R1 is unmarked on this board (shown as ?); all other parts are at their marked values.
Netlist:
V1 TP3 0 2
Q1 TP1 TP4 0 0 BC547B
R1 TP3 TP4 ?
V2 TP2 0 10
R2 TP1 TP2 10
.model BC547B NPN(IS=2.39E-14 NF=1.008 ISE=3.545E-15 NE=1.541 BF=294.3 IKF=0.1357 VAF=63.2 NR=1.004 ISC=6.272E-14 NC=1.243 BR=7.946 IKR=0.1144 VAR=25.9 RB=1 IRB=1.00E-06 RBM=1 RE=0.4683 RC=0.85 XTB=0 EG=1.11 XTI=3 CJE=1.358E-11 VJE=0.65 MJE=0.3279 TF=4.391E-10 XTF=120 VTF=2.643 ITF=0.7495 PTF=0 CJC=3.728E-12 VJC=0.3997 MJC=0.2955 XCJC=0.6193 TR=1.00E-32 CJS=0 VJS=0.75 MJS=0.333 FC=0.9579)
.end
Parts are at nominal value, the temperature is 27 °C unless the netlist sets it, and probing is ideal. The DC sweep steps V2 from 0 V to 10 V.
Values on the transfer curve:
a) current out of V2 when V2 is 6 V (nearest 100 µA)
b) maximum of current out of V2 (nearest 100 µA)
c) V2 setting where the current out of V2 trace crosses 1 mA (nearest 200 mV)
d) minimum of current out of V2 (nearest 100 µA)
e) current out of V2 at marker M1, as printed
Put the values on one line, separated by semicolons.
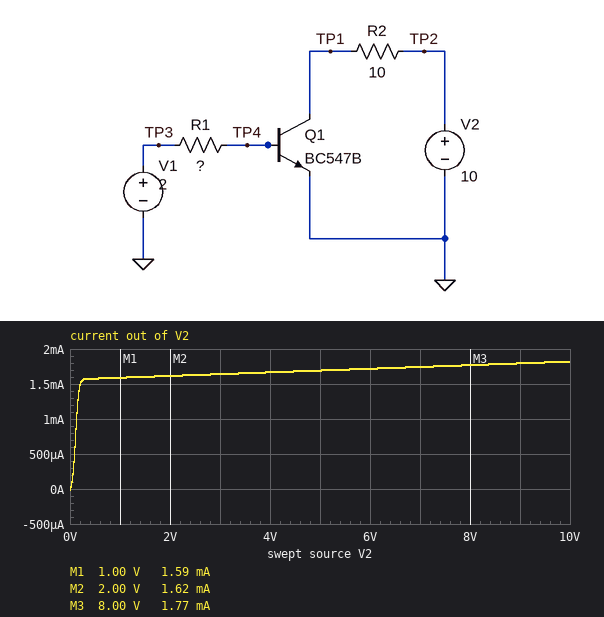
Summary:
1.7 mA; 1.8 mA; 200 mV; 0 A; 1.59 mA
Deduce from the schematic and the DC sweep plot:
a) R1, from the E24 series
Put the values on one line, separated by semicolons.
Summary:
240 kΩ
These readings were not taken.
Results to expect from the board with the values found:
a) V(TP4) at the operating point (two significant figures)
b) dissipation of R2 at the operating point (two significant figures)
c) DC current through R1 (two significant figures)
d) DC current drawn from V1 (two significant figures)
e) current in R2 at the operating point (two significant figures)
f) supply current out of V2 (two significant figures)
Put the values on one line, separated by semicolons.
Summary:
650 mV; 33 µW; 5.6 µA; 5.6 µA; 1.8 mA; 1.8 mA
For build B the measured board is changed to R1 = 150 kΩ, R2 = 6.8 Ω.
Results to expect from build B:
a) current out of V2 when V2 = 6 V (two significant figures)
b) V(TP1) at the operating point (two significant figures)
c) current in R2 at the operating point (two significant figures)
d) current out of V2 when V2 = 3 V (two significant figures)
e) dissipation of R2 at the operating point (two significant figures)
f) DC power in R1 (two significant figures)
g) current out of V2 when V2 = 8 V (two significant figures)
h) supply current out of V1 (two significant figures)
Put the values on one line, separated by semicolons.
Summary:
2.7 mA; 10 V; 2.9 mA; 2.6 mA; 56 µW; 12 µW; 2.8 mA; 8.9 µA
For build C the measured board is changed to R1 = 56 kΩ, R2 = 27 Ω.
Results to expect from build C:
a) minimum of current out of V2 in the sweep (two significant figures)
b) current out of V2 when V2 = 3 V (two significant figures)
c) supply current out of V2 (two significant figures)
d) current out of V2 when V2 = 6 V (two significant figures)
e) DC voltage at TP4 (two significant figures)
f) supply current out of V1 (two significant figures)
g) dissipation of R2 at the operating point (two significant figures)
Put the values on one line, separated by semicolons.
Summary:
-33 µA; 6.6 mA; 7.3 mA; 6.9 mA; 690 mV; 23 µA; 1.4 mW
